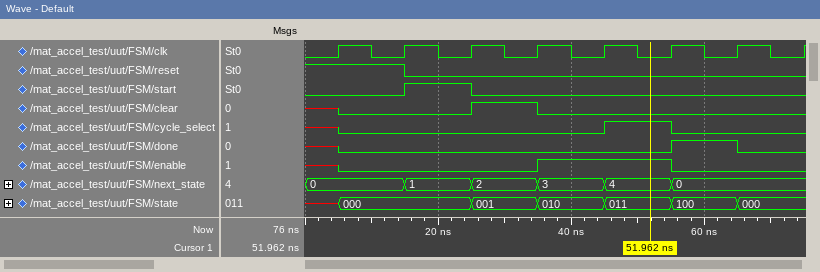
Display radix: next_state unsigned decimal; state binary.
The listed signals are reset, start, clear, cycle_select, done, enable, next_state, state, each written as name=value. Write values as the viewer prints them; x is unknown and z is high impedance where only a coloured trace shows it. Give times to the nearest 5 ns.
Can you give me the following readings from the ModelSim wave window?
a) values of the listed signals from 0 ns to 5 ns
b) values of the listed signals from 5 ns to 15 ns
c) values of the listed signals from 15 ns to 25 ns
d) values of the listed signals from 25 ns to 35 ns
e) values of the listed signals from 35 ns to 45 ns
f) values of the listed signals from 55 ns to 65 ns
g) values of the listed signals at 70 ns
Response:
reset=1, start=0, clear=x, cycle_select=x, done=x, enable=x, next_state=0, state=x
reset=1, start=0, clear=0, cycle_select=0, done=0, enable=0, next_state=0, state=000
reset=0, start=1, clear=0, cycle_select=0, done=0, enable=0, next_state=1, state=000
reset=0, start=0, clear=1, cycle_select=0, done=0, enable=0, next_state=2, state=001
reset=0, start=0, clear=0, cycle_select=0, done=0, enable=1, next_state=3, state=010
reset=0, start=0, clear=0, cycle_select=0, done=1, enable=0, next_state=0, state=100
reset=0, start=0, clear=0, cycle_select=0, done=0, enable=0, next_state=0, state=000
